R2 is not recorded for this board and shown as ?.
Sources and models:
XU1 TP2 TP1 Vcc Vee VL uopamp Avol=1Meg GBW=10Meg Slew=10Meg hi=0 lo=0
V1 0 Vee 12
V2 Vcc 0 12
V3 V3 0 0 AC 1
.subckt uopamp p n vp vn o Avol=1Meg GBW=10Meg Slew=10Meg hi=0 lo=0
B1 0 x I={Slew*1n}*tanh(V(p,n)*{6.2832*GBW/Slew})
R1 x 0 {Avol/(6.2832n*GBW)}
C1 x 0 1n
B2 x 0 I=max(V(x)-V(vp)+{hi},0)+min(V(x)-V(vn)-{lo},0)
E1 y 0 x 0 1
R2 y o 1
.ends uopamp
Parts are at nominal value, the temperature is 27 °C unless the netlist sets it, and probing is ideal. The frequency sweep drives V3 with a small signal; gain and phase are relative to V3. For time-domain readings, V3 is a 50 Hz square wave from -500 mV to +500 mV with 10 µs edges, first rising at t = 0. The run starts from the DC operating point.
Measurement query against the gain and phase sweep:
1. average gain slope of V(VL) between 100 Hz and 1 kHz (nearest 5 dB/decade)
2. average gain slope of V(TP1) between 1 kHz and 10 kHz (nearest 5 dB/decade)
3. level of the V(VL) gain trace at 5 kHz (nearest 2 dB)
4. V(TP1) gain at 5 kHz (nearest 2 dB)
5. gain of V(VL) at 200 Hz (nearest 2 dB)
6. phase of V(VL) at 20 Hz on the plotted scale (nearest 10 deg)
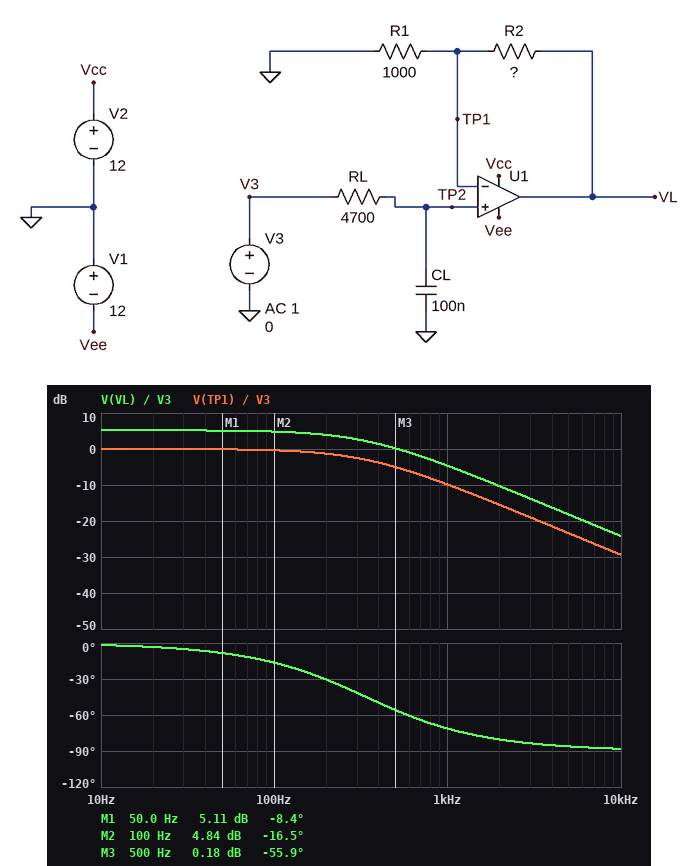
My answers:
-10 dB/decade
-20 dB/decade
-18 dB
-24 dB
4 dB
0 deg
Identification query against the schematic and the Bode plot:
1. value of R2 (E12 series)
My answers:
820 Ω
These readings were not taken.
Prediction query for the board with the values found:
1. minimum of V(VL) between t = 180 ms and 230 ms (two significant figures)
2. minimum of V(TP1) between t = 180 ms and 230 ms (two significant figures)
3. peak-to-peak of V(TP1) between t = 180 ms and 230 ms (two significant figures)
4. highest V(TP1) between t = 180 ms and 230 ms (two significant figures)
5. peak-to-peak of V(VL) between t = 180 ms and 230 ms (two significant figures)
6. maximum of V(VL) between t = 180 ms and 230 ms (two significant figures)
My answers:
-910 mV
-500 mV
1.0 V
500 mV
1.8 V
910 mV
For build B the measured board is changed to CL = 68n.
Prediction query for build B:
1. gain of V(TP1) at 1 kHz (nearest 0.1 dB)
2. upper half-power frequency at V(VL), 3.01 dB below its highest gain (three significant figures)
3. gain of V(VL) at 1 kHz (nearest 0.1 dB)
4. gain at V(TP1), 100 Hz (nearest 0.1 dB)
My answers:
-7.0 dB
498 Hz
-1.8 dB
-0.2 dB
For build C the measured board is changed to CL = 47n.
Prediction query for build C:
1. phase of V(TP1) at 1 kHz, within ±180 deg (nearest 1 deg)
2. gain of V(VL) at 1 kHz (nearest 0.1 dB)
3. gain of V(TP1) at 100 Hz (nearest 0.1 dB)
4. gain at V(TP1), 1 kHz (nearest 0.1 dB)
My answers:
-54 deg
0.5 dB
-0.1 dB
-4.7 dB
